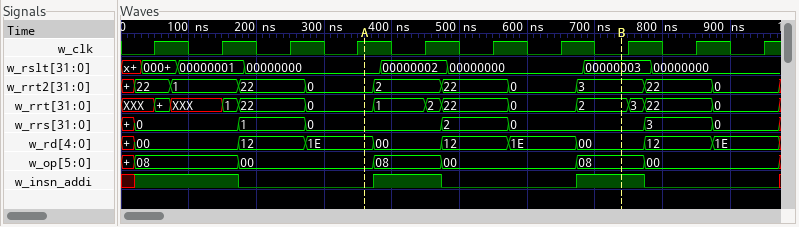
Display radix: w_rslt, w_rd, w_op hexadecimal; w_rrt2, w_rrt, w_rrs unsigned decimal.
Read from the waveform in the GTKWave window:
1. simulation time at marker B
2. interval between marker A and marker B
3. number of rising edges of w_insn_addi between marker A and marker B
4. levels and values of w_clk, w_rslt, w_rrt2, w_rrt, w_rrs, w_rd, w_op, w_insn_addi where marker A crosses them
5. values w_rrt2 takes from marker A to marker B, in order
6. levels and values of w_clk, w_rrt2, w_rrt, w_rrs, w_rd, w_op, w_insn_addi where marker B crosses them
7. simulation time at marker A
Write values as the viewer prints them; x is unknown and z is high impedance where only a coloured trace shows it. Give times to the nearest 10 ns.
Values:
740 ns
380 ns
2
w_clk=1, w_rslt=00000000, w_rrt2=0, w_rrt=0, w_rrs=0, w_rd=1E, w_op=00, w_insn_addi=0
0, 2, 22, 0, 3
w_clk=0, w_rrt2=3, w_rrt=2, w_rrs=0, w_rd=00, w_op=08, w_insn_addi=1
360 ns
